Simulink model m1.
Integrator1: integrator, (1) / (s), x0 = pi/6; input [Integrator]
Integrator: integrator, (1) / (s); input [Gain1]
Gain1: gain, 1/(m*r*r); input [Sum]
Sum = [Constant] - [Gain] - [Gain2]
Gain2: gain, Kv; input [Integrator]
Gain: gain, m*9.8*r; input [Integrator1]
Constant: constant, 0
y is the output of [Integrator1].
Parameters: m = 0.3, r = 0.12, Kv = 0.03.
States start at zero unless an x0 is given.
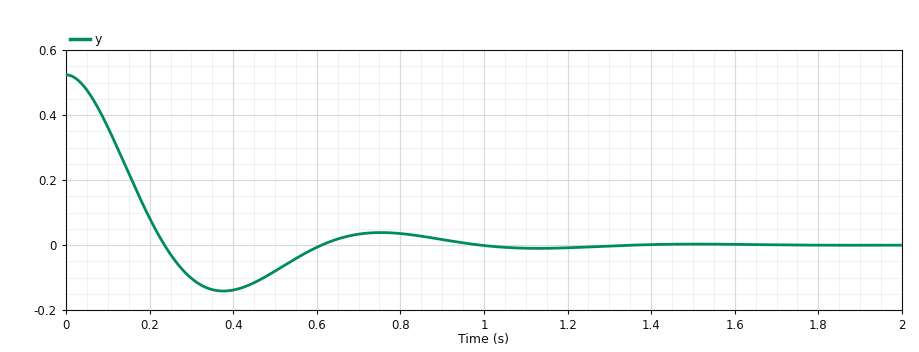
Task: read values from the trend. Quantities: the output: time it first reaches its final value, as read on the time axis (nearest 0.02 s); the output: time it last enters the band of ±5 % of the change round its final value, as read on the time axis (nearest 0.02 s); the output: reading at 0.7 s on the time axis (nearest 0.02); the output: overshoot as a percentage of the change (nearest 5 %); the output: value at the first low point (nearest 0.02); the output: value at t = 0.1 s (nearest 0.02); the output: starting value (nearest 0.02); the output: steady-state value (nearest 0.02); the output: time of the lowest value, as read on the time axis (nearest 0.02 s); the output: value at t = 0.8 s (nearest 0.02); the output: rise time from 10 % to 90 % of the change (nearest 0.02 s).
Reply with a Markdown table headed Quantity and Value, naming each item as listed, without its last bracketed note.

| Quantity | Value |
|---|---|
| the output: time it first reaches its final value, as read on the time axis | 0.24 s |
| the output: time it last enters the band of ±5 % of the change round its final value, as read on the time axis | 0.86 s |
| the output: reading at 0.7 s on the time axis | 0.04 |
| the output: overshoot as a percentage of the change | 25 % |
| the output: value at the first low point | -0.14 |
| the output: value at t = 0.1 s | 0.36 |
| the output: starting value | 0.52 |
| the output: steady-state value | 0.00 |
| the output: time of the lowest value, as read on the time axis | 0.38 s |
| the output: value at t = 0.8 s | 0.04 |
| the output: rise time from 10 % to 90 % of the change | 0.16 s |
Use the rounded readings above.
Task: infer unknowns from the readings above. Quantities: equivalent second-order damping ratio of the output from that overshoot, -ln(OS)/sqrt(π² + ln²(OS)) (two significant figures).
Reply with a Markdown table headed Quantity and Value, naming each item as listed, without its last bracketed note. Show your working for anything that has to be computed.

| Quantity | Value |
|---|---|
| equivalent second-order damping ratio of the output from that overshoot, -ln(OS)/sqrt(π² + ln²(OS)) | ln(0.25) = -1.386; 1.386 / sqrt(9.870 + 1.922) = 0.40 |
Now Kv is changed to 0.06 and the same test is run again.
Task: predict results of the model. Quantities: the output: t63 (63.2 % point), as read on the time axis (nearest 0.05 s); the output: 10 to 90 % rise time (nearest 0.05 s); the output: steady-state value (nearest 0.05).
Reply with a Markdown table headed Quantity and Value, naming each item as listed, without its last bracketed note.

| Quantity | Value |
|---|---|
| the output: t63 (63.2 % point), as read on the time axis | 0.20 s |
| the output: 10 to 90 % rise time | 0.25 s |
| the output: steady-state value | 0.00 |
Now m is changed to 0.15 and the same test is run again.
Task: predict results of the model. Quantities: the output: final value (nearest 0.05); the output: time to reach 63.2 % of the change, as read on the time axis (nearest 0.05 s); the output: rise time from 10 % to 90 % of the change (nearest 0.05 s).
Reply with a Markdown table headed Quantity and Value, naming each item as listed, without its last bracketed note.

| Quantity | Value |
|---|---|
| the output: final value | 0.00 |
| the output: time to reach 63.2 % of the change, as read on the time axis | 0.20 s |
| the output: rise time from 10 % to 90 % of the change | 0.25 s |
